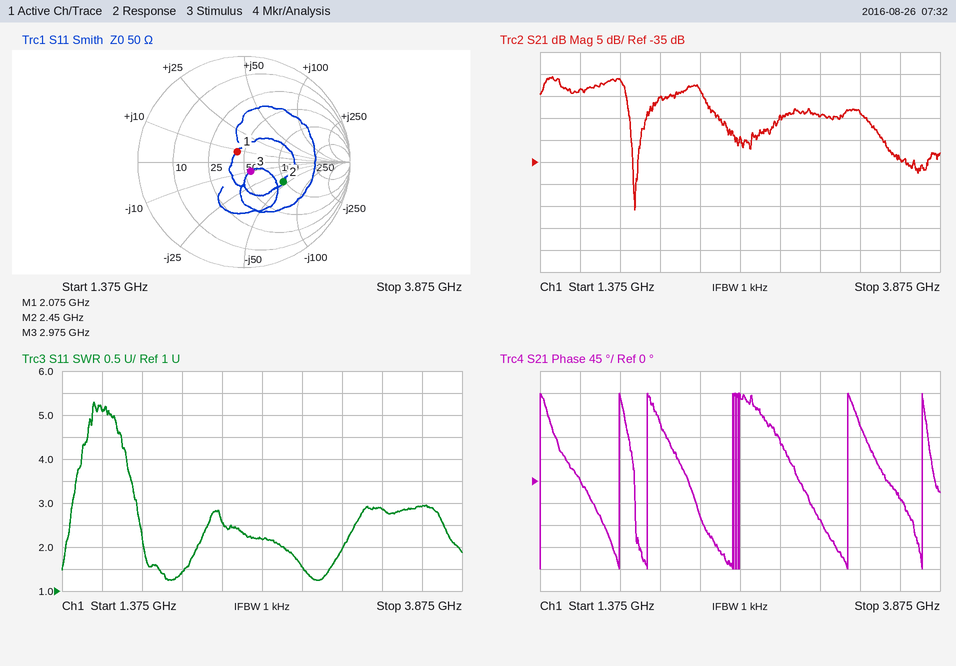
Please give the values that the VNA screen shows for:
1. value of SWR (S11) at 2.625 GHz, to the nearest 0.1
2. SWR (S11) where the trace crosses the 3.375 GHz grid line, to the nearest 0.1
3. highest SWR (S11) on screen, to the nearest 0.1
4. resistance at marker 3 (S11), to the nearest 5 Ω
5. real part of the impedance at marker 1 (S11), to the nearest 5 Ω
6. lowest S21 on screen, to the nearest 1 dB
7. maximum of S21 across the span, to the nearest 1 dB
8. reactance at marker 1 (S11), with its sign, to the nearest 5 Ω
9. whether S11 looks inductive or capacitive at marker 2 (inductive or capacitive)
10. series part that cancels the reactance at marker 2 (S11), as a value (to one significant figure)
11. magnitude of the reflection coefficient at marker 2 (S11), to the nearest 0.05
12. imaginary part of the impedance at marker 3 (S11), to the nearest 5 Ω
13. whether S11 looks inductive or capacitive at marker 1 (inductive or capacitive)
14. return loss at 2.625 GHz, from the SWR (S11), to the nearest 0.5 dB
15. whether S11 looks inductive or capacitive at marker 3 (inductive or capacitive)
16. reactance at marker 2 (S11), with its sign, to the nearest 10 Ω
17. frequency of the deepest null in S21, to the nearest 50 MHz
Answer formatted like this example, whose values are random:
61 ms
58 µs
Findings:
2.2
2.9
5.3
55 Ω
45 Ω
-46 dB
-16 dB
+10 Ω
capacitive
3 nH
0.40
-10 Ω
inductive
8.5 dB
capacitive
-40 Ω
1.95 GHz
